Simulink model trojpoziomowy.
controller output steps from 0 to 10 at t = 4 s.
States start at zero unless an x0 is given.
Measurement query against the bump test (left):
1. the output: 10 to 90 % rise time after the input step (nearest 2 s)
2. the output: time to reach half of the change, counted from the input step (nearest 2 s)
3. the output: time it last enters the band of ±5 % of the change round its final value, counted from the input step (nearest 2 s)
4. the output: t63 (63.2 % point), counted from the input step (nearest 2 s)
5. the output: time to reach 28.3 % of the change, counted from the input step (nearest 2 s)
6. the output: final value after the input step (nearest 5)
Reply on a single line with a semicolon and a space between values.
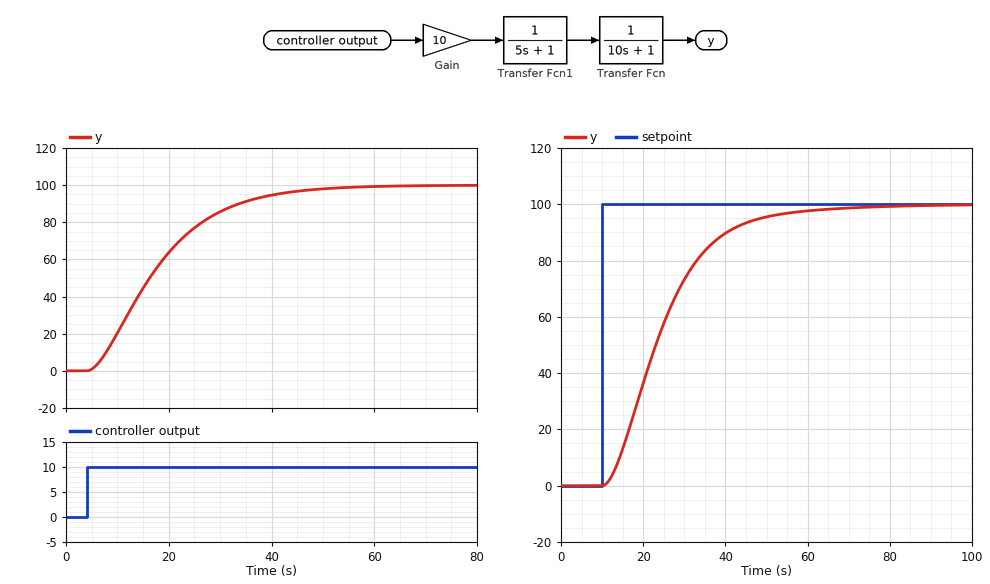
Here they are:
26 s; 12 s; 36 s; 16 s; 8 s; 100
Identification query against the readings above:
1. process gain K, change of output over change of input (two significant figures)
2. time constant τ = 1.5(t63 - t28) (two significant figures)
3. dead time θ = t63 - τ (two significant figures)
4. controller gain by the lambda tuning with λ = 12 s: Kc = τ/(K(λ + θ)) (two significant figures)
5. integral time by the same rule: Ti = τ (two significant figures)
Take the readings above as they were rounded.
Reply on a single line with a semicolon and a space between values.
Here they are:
10; 12 s; 4.0 s; 0.075; 12 s
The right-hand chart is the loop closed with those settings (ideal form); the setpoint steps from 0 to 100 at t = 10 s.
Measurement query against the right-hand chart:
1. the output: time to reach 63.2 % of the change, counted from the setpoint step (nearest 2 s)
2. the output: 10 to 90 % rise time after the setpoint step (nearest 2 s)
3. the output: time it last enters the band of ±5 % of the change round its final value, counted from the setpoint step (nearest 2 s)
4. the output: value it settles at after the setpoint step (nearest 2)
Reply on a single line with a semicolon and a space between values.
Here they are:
16 s; 26 s; 38 s; 100
